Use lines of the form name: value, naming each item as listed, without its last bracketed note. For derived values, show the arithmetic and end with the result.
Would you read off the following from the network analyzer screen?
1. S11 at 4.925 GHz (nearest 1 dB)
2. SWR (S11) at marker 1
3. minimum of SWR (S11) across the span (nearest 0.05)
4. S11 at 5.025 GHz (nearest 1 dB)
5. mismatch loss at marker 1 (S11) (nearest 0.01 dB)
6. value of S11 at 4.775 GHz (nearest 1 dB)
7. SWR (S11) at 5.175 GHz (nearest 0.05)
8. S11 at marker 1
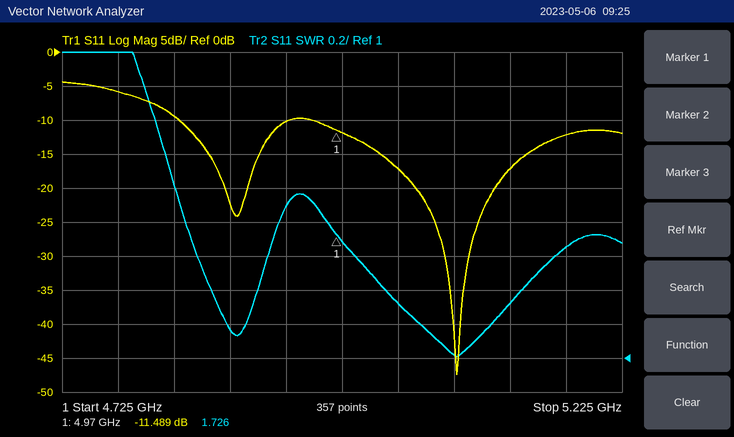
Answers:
S11 at 4.925 GHz: -10 dB
SWR (S11) at marker 1: 1.726
minimum of SWR (S11) across the span: 1.00
S11 at 5.025 GHz: -17 dB
mismatch loss at marker 1 (S11): −10 log10(1 − 10^(-11.489/10)) ≈ 0.32 dB
value of S11 at 4.775 GHz: -6 dB
SWR (S11) at 5.175 GHz: 1.65
S11 at marker 1: -11.489 dB
